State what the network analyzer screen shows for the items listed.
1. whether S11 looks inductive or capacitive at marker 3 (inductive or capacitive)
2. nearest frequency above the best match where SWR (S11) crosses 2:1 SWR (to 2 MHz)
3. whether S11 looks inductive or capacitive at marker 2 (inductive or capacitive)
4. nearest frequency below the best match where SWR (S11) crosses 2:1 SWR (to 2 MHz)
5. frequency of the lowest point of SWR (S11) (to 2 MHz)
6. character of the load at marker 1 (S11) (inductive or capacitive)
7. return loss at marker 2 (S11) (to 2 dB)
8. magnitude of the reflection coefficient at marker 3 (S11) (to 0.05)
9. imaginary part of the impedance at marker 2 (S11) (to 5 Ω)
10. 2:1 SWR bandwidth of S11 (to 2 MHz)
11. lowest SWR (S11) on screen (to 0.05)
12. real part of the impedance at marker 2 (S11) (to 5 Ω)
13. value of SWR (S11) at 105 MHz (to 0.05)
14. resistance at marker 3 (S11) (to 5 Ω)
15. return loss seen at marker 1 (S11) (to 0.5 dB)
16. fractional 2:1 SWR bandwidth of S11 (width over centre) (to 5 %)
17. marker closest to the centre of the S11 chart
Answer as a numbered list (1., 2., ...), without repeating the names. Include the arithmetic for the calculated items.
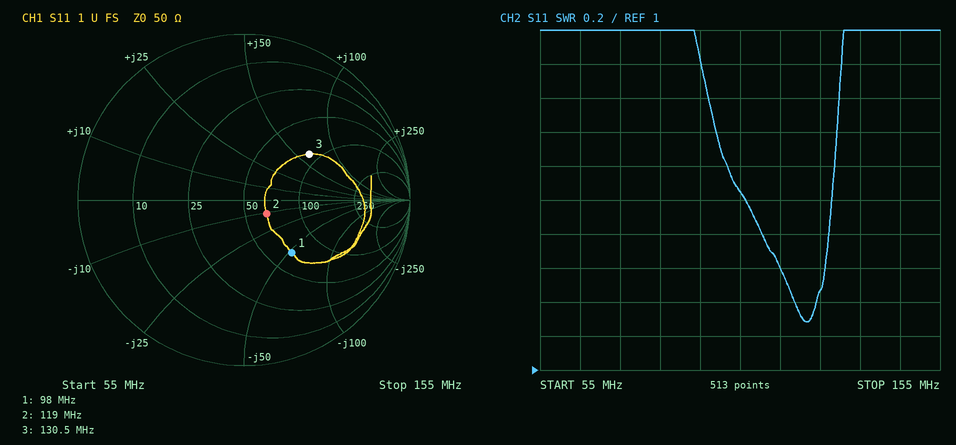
1. inductive
2. 128 MHz
3. capacitive
4. 106 MHz
5. 122 MHz
6. capacitive
7. 16 dB
8. 0.50
9. -10 Ω
10. 128 MHz − 106 MHz = 22 MHz
11. 1.30
12. 65 Ω
13. 2.05
14. 85 Ω
15. 7.5 dB
16. 22 MHz / 117 MHz ≈ 18.8 %, so 20 % to the nearest 5 %
17. marker 2
